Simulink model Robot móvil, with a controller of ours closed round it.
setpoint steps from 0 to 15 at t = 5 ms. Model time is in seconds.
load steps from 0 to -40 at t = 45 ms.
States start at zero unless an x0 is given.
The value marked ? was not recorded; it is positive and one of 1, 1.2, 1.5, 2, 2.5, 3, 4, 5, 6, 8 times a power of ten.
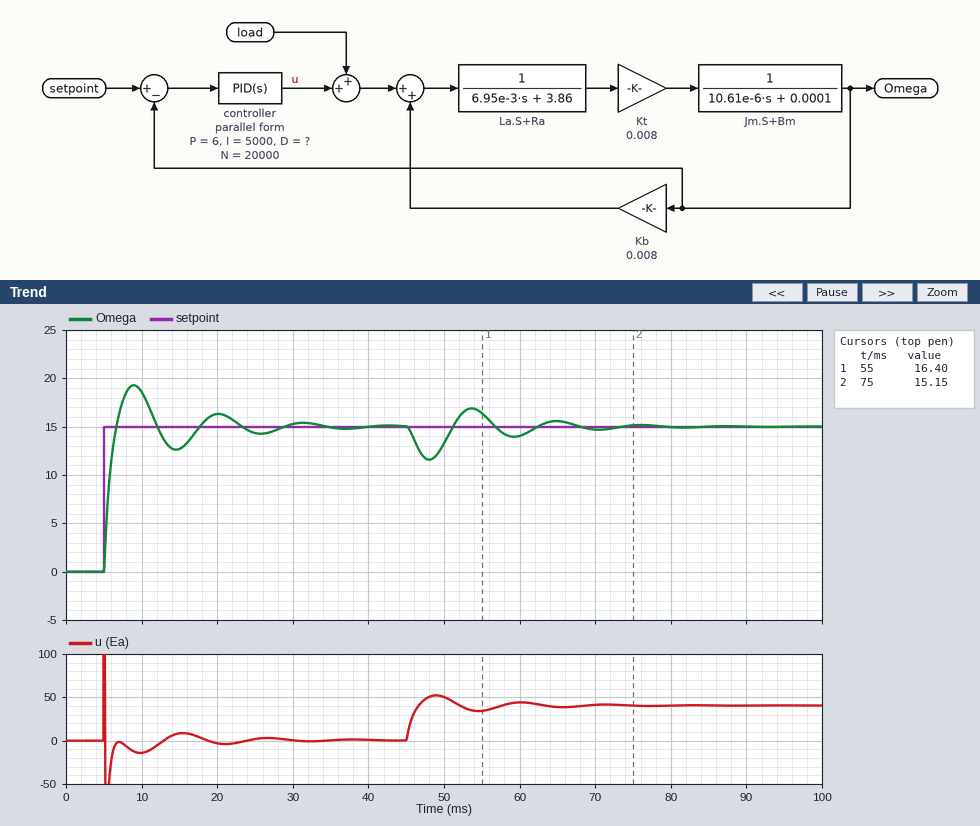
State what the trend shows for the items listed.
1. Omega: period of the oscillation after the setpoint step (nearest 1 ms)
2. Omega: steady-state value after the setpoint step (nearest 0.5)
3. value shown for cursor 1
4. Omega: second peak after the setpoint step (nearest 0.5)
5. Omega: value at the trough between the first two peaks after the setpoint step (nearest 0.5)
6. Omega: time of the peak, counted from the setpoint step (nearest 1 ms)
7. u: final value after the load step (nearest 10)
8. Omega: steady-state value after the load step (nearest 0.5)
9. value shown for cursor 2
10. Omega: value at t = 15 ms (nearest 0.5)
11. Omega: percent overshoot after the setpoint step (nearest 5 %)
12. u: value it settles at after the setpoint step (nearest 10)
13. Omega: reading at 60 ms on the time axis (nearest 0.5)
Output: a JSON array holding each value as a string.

["11 ms", "15.0", "16.40", "16.5", "12.5", "4 ms", "40", "15.0", "15.15", "12.5", "30 %", "0", "14.0"]
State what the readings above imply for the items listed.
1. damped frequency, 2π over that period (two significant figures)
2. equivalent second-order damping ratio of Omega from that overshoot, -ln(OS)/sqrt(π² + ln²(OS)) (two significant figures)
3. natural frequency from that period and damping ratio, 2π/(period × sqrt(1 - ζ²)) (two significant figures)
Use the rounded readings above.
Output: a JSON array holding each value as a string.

["0.57 rad/ms", "0.36", "0.61 rad/ms"]
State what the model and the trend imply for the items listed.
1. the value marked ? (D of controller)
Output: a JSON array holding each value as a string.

["0.012"]
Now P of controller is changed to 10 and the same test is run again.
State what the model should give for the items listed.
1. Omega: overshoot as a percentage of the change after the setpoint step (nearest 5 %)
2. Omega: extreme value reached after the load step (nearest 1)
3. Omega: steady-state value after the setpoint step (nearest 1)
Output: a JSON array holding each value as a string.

["25 %", "12", "15"]
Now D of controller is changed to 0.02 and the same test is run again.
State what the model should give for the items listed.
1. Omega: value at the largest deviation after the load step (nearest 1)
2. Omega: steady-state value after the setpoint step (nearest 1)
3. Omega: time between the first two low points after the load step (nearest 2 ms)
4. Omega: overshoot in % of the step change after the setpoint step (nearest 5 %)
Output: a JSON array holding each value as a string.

["12", "15", "14 ms", "15 %"]
